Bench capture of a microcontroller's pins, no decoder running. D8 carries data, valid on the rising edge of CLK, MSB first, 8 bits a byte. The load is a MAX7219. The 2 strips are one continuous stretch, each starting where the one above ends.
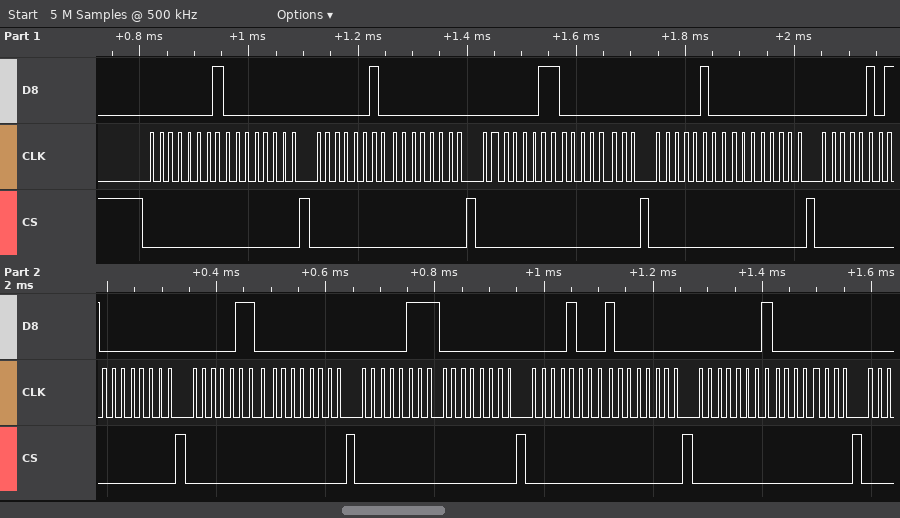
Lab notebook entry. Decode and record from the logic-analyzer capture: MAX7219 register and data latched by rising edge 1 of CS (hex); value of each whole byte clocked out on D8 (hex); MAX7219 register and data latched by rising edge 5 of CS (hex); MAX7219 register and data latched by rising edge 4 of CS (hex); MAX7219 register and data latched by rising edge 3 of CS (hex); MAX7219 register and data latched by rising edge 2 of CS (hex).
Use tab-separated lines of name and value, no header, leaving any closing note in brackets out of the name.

MAX7219 register and data latched by rising edge 1 of CS	register 0x1, data 0x00
value of each whole byte clocked out on D8	01 00 02 00 03 00 04 00 05 00 06 00 07 00 08 80 01 00
MAX7219 register and data latched by rising edge 5 of CS	register 0x5, data 0x00
MAX7219 register and data latched by rising edge 4 of CS	register 0x4, data 0x00
MAX7219 register and data latched by rising edge 3 of CS	register 0x3, data 0x00
MAX7219 register and data latched by rising edge 2 of CS	register 0x2, data 0x00
